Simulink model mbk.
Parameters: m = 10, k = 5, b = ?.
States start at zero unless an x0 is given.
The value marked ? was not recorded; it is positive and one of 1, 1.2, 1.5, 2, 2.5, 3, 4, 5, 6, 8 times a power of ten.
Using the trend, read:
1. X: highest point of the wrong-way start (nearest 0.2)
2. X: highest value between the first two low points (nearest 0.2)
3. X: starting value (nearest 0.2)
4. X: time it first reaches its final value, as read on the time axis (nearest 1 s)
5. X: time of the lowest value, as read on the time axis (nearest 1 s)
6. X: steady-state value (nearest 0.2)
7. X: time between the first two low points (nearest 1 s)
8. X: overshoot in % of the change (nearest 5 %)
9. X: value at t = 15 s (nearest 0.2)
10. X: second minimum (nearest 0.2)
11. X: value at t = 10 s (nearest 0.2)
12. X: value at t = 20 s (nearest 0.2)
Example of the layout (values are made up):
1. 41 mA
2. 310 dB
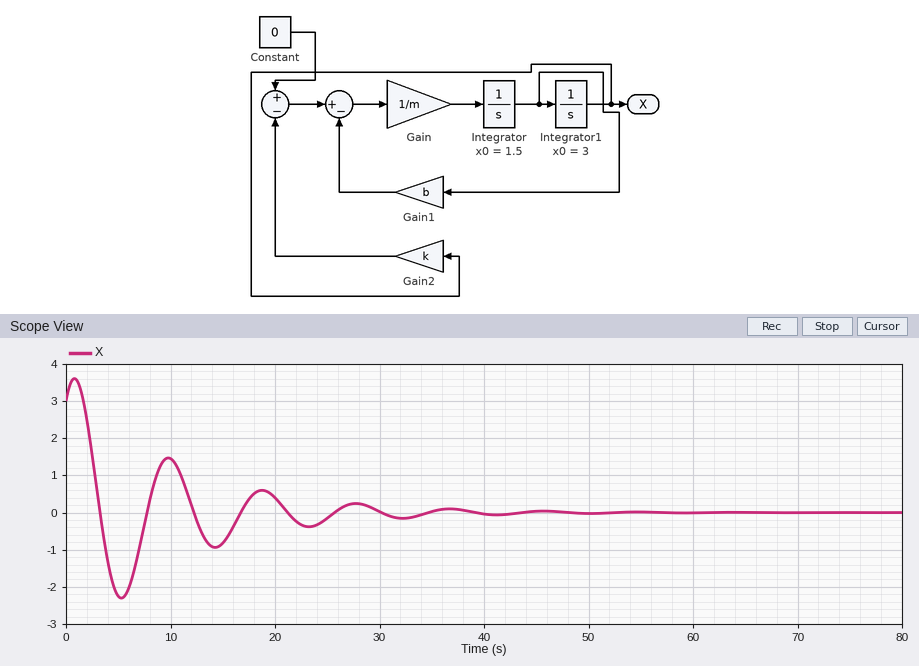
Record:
1. 3.6
2. 1.4
3. 3.0
4. 3 s
5. 5 s
6. 0.0
7. 9 s
8. 75 %
9. -0.8
10. -1.0
11. 1.4
12. 0.4
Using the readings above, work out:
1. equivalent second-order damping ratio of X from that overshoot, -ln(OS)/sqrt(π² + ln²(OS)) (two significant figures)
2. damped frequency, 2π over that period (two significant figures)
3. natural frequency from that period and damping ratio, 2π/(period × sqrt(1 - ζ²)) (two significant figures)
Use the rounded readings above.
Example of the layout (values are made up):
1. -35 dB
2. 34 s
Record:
1. 0.091
2. 0.70 rad/s
3. 0.70 rad/s
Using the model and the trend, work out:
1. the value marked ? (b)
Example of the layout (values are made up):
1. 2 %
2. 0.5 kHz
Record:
1. 2
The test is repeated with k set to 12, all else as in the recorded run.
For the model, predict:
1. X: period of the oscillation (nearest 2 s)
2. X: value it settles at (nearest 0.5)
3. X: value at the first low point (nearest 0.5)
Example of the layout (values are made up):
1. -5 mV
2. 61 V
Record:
1. 6 s
2. 0.0
3. -2.5
